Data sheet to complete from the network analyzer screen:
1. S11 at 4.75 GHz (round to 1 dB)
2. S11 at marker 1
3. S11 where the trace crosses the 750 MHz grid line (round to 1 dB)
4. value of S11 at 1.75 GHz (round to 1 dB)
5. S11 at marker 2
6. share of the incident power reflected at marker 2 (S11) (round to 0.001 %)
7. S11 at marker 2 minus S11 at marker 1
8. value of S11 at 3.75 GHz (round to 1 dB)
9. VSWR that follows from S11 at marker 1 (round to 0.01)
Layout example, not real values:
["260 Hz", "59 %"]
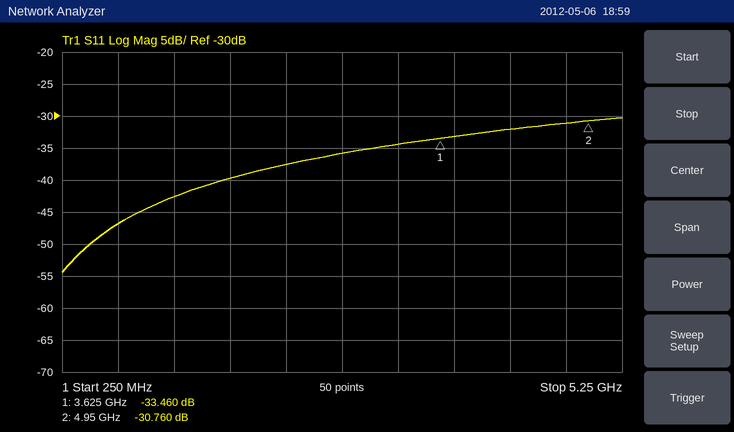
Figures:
["-31 dB", "-33.460 dB", "-47 dB", "-40 dB", "-30.760 dB", "0.084 %", "2.700 dB", "-33 dB", "1.04"]
